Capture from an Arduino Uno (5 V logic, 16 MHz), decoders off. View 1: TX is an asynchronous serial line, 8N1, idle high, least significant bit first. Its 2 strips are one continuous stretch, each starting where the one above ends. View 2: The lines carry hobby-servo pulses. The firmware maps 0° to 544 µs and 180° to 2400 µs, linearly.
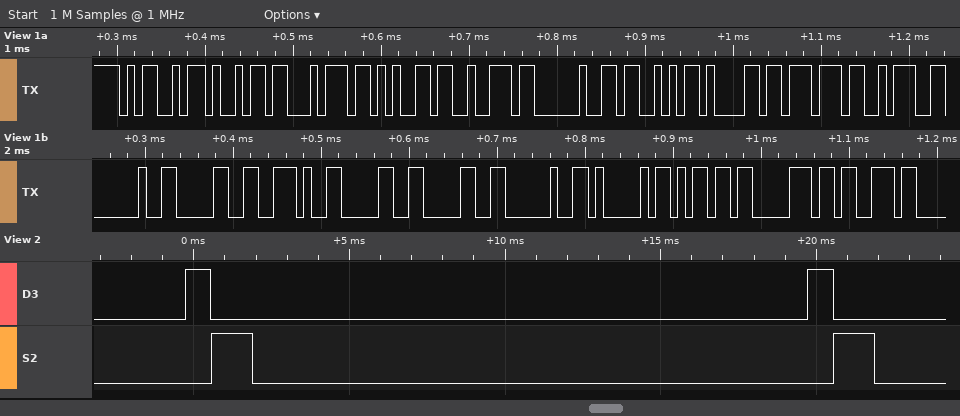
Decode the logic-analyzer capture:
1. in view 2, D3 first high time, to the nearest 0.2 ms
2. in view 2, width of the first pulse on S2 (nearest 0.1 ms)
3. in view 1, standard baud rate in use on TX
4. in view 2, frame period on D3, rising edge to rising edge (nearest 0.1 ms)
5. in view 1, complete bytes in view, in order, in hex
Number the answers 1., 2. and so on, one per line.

1. 0.8 ms
2. 1.3 ms
3. 115200 baud
4. 20.0 ms
5. 0x4D 0x69 0x74 0x65 0x72 0x20 0x53 0x61 0x77 0x3A 0x20 0x30 0x2E 0x30 0x30 0x20 0x41 0x6D 0x70 0x73
